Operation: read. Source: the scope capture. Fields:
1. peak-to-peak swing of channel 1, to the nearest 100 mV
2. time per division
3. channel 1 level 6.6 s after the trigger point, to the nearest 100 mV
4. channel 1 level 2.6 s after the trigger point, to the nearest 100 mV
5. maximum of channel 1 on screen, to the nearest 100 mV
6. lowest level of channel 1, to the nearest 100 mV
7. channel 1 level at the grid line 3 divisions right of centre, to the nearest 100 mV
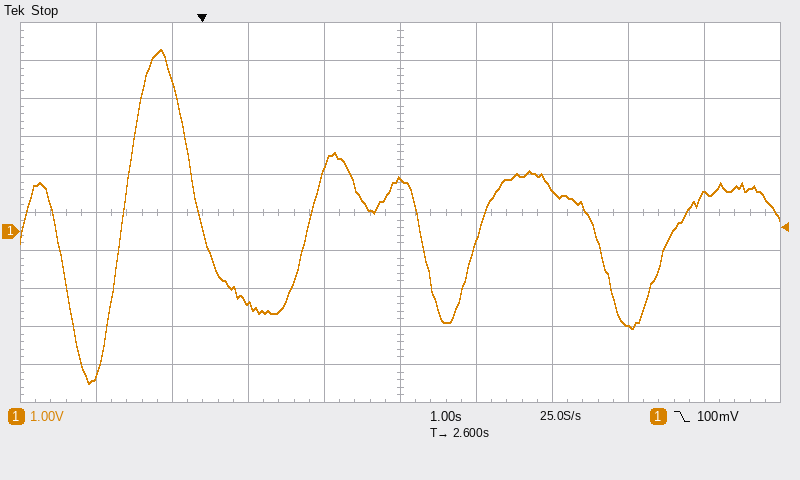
8.8 V
1 s
1.0 V
1.4 V
4.8 V
-4.0 V
-2.5 V
